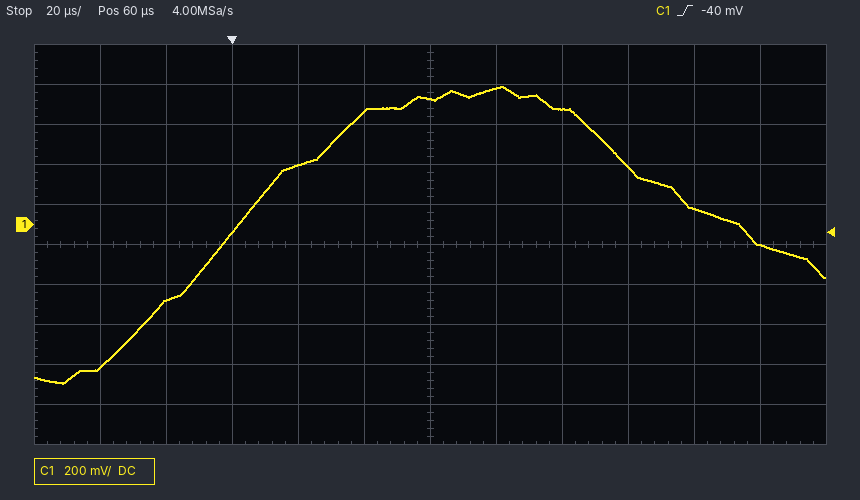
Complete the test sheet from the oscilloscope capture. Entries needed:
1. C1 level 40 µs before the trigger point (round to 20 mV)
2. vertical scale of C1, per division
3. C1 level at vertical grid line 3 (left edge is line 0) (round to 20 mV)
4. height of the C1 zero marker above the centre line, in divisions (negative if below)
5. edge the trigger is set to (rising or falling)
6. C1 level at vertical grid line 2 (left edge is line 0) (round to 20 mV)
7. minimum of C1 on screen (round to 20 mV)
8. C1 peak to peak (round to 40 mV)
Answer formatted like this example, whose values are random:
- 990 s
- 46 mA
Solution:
- -720 mV
- 200 mV
- -40 mV
- +0.5 div
- rising
- -380 mV
- -800 mV
- 1.48 V
